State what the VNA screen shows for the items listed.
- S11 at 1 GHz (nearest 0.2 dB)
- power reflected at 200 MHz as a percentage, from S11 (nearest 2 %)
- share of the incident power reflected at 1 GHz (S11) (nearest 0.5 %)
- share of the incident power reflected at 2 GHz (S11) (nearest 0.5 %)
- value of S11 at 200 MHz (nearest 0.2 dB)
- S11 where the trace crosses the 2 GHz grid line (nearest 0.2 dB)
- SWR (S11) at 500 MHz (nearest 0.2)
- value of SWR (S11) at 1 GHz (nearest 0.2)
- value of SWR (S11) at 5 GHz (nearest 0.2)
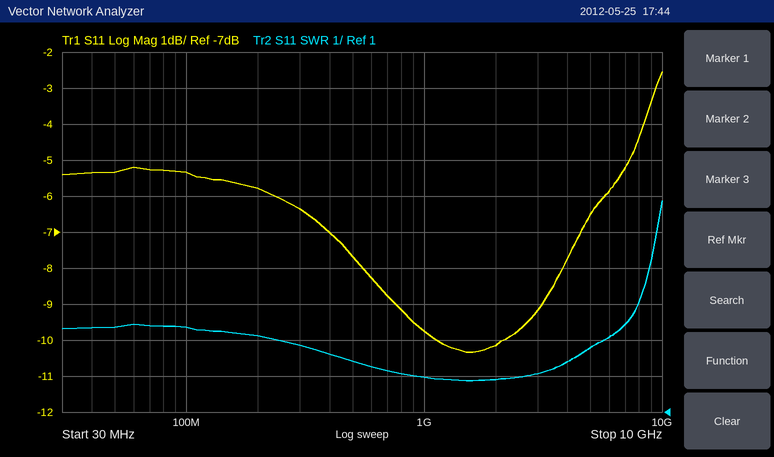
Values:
-9.8 dB
26 %
10.5 %
9.5 %
-5.8 dB
-10.2 dB
2.4
2.0
2.8
